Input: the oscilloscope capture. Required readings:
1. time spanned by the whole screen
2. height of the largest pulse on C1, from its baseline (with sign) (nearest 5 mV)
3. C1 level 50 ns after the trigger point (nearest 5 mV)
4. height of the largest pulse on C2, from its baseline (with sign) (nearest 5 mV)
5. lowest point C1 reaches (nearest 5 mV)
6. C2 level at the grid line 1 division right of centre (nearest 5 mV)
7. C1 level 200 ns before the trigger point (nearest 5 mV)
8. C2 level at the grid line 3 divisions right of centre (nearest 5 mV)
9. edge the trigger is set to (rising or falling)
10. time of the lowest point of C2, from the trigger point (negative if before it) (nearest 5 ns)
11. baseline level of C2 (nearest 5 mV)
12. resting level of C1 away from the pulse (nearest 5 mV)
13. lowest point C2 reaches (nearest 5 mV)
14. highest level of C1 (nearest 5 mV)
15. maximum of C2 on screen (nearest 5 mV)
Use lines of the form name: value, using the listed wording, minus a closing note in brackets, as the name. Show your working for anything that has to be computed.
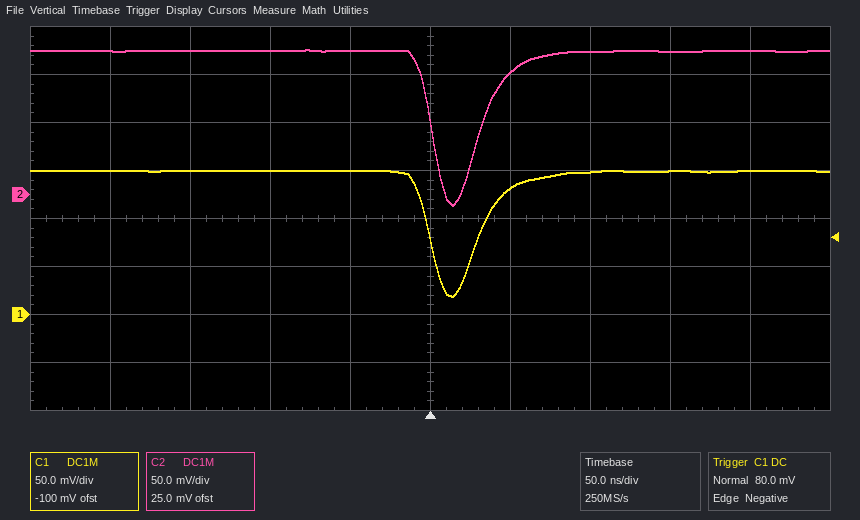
time spanned by the whole screen: 500 ns
height of the largest pulse on C1, from its baseline (with sign): 20 mV − (150 mV) = -130 mV
C1 level 50 ns after the trigger point: 130 mV
height of the largest pulse on C2, from its baseline (with sign): -10 mV − (150 mV) = -160 mV
lowest point C1 reaches: 20 mV
C2 level at the grid line 1 division right of centre: 125 mV
C1 level 200 ns before the trigger point: 150 mV
C2 level at the grid line 3 divisions right of centre: 150 mV
edge the trigger is set to: falling
time of the lowest point of C2, from the trigger point (negative if before it): +15 ns
baseline level of C2: 150 mV
resting level of C1 away from the pulse: 150 mV
lowest point C2 reaches: -10 mV
highest level of C1: 150 mV
maximum of C2 on screen: 150 mV
